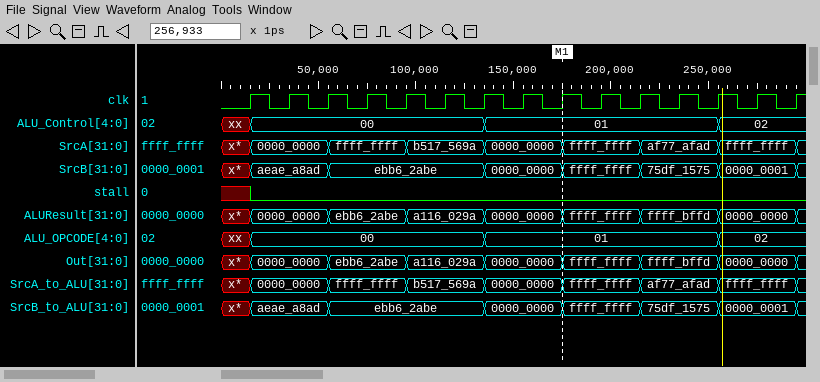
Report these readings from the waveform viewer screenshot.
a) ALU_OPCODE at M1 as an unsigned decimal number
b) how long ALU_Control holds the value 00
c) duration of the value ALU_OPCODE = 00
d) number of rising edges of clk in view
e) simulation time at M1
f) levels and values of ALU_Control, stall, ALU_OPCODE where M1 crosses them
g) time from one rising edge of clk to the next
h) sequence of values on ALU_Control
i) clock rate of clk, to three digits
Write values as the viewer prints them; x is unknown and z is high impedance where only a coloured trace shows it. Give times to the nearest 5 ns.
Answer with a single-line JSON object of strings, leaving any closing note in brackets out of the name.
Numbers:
{"ALU_OPCODE at M1 as an unsigned decimal number": "1", "how long ALU_Control holds the value 00": "120 ns", "duration of the value ALU_OPCODE = 00": "120 ns", "number of rising edges of clk in view": "15", "simulation time at M1": "175 ns", "levels and values of ALU_Control, stall, ALU_OPCODE where M1 crosses them": "ALU_Control=01, stall=0, ALU_OPCODE=01", "time from one rising edge of clk to the next": "20 ns", "sequence of values on ALU_Control": "xx, 00, 01, 02", "clock rate of clk, to three digits": "50.0 MHz"}
